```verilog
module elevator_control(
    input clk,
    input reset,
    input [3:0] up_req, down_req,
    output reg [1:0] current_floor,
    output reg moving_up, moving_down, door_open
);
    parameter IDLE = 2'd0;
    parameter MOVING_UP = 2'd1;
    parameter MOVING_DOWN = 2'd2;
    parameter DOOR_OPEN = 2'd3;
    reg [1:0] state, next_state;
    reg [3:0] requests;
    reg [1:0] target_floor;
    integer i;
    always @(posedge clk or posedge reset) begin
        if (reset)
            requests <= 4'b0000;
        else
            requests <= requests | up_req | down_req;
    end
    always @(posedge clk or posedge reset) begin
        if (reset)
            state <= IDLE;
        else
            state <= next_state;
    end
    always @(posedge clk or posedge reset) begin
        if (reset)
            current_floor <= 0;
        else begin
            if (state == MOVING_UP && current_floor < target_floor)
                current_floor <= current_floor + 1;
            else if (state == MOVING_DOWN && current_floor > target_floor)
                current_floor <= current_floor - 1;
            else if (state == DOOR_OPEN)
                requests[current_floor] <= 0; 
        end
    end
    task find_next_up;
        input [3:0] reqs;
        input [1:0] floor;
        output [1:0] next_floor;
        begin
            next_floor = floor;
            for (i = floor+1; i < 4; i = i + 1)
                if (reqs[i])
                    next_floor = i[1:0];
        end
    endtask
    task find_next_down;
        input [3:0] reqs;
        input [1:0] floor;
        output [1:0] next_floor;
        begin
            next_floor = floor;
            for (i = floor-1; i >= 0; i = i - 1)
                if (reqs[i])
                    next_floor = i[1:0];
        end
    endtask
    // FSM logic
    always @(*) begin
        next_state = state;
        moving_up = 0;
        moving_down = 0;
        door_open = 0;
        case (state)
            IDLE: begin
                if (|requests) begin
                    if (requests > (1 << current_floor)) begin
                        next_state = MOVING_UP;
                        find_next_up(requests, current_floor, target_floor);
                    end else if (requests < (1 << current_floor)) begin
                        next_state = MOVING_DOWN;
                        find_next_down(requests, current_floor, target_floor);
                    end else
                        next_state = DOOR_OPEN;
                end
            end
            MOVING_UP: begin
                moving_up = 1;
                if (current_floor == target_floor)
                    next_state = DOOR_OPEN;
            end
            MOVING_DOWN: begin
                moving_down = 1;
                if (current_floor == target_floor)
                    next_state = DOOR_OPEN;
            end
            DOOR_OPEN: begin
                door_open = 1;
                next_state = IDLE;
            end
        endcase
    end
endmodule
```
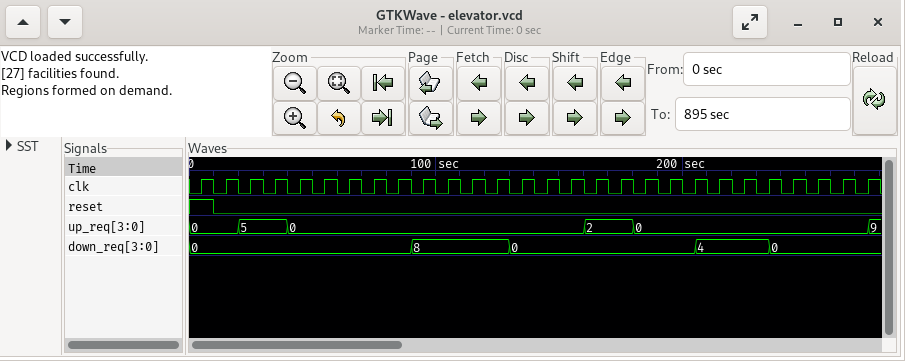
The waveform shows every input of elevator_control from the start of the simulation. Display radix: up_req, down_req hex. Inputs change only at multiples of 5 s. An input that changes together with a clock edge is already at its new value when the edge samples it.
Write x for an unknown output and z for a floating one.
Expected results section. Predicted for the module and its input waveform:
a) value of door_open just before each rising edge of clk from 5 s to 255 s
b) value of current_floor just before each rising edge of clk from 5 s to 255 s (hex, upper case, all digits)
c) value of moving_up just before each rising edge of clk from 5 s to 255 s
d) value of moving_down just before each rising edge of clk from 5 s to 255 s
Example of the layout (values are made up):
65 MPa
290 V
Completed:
0 0 0 0 0 0 0 1 0 0 1 0 0 0 1 0 0 0 0 0 1 0 0 0 0 1
0, 0, 0, 0, 0, 1, 2, 2, 2, 2, 2, 2, 2, 3, 3, 3, 3, 2, 1, 0, 0, 0, 0, 1, 2, 2
0 0 0 0 1 1 1 0 0 1 0 0 1 1 0 0 0 0 0 0 0 0 1 1 1 0
0 0 0 0 0 0 0 0 0 0 0 0 0 0 0 0 1 1 1 1 0 0 0 0 0 0
